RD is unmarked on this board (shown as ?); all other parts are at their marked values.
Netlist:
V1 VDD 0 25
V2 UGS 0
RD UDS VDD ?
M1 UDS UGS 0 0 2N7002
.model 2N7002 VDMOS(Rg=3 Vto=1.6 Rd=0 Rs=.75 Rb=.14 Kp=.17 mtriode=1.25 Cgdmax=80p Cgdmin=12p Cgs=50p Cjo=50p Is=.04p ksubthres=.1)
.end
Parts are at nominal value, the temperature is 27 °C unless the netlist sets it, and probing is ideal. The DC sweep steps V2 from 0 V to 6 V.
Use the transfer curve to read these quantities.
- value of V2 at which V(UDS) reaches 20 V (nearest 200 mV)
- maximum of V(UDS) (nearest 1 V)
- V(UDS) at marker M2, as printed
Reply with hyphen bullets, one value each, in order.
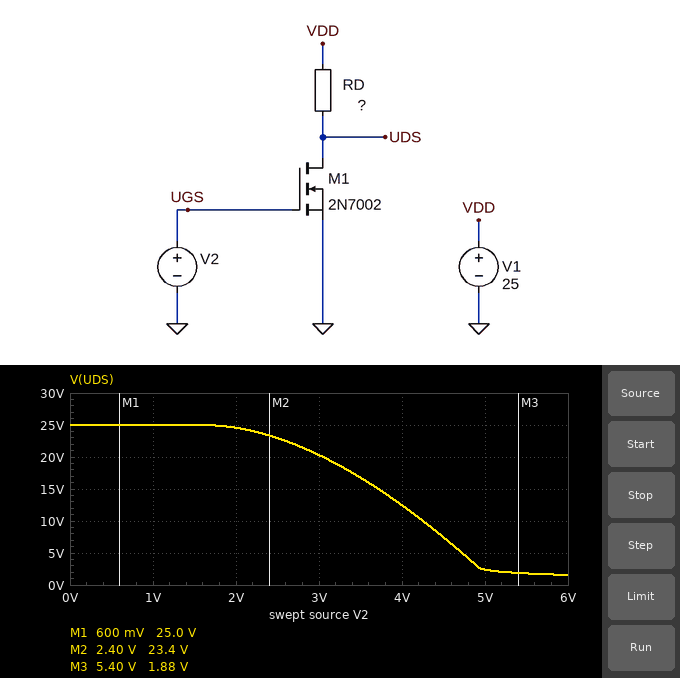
- 3.0 V
- 25 V
- 23.4 V
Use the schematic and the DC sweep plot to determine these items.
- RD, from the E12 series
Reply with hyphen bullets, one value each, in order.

- 33 Ω
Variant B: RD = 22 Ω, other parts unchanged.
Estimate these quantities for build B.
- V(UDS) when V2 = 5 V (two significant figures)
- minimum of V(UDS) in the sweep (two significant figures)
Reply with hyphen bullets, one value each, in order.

- 9.6 V
- 2.7 V
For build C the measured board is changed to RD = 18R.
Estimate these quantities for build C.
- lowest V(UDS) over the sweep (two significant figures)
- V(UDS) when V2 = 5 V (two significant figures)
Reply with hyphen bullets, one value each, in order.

- 5.4 V
- 12 V
